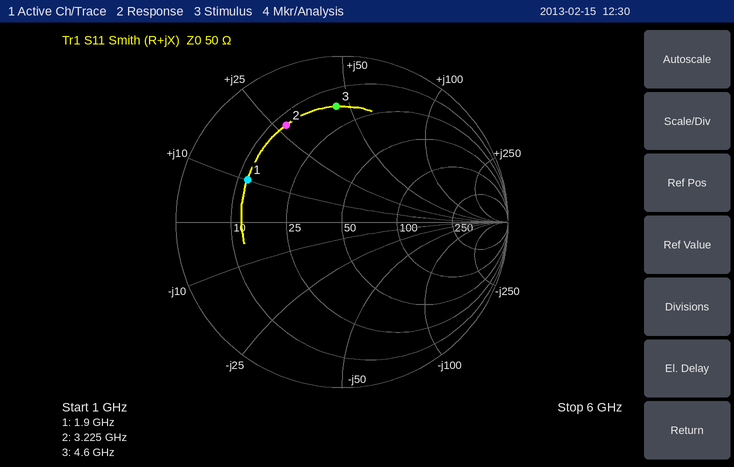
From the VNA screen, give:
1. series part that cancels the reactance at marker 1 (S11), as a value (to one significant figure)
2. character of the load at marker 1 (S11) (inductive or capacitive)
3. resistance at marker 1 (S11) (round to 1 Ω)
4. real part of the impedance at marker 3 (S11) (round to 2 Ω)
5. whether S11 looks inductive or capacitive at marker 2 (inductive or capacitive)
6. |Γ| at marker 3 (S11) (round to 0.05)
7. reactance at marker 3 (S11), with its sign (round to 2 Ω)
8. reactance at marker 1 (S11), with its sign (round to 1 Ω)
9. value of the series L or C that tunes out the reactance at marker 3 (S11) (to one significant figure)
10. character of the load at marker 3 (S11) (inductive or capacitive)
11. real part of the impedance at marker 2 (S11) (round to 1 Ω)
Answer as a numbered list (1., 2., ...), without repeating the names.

1. 8 pF
2. inductive
3. 12 Ω
4. 16 Ω
5. inductive
6. 0.70
7. +44 Ω
8. +10 Ω
9. 800 fF
10. inductive
11. 13 Ω
